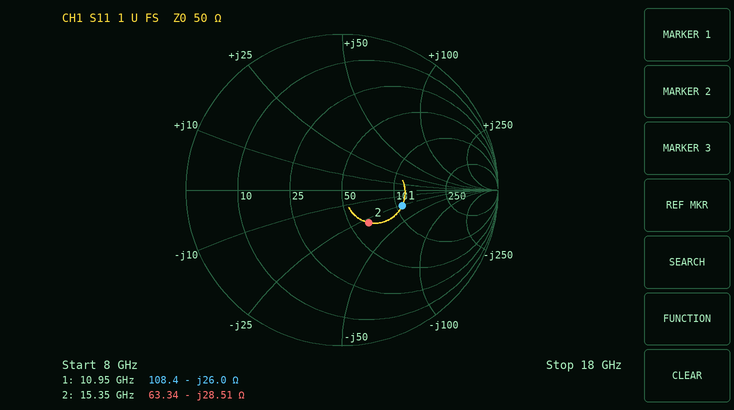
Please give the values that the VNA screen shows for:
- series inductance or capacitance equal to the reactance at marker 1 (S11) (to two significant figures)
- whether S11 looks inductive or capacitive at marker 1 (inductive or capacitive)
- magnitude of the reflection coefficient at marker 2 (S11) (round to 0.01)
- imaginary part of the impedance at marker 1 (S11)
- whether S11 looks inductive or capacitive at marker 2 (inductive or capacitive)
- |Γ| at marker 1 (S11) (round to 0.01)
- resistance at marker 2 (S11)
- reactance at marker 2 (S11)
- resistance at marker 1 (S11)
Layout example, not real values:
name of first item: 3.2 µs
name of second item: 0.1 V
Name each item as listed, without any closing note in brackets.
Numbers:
series inductance or capacitance equal to the reactance at marker 1 (S11): 560 fF
whether S11 looks inductive or capacitive at marker 1: capacitive
magnitude of the reflection coefficient at marker 2 (S11): 0.27
imaginary part of the impedance at marker 1: -26.0 Ω
whether S11 looks inductive or capacitive at marker 2: capacitive
|Γ| at marker 1 (S11): 0.40
resistance at marker 2: 63.34 Ω
reactance at marker 2: -28.51 Ω
resistance at marker 1: 108.4 Ω
